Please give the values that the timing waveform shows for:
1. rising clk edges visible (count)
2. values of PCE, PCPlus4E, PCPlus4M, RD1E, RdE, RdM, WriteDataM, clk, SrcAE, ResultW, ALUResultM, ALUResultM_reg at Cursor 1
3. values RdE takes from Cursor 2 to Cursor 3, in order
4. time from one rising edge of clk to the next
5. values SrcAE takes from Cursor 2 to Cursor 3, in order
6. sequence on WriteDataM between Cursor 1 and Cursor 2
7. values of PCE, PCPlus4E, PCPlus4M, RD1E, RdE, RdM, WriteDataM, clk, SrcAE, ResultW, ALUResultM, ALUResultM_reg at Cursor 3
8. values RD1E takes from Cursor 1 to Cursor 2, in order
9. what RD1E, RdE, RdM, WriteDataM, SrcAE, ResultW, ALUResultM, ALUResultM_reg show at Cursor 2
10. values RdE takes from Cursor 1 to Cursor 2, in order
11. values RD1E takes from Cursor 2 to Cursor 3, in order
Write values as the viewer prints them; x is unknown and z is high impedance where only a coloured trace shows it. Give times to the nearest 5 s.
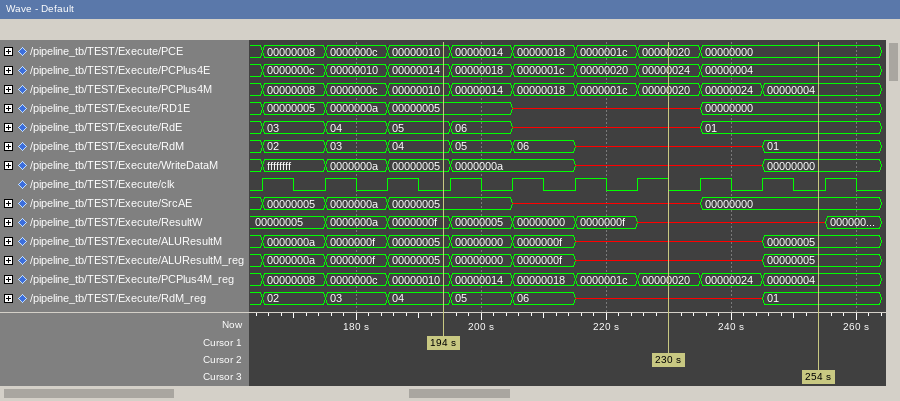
10
PCE=00000010, PCPlus4E=00000014, PCPlus4M=00000010, RD1E=00000005, RdE=05, RdM=04, WriteDataM=00000005, clk=0, SrcAE=00000005, ResultW=0000000f, ALUResultM=00000005, ALUResultM_reg=00000005
x, 01
10 s
x, 00000000
00000005, 0000000a, x
PCE=00000000, PCPlus4E=00000004, PCPlus4M=00000004, RD1E=00000000, RdE=01, RdM=01, WriteDataM=00000000, clk=0, SrcAE=00000000, ResultW=x, ALUResultM=00000005, ALUResultM_reg=00000005
00000005, x
RD1E=x, RdE=x, RdM=x, WriteDataM=x, SrcAE=x, ResultW=x, ALUResultM=x, ALUResultM_reg=x
05, 06, x
x, 00000000
